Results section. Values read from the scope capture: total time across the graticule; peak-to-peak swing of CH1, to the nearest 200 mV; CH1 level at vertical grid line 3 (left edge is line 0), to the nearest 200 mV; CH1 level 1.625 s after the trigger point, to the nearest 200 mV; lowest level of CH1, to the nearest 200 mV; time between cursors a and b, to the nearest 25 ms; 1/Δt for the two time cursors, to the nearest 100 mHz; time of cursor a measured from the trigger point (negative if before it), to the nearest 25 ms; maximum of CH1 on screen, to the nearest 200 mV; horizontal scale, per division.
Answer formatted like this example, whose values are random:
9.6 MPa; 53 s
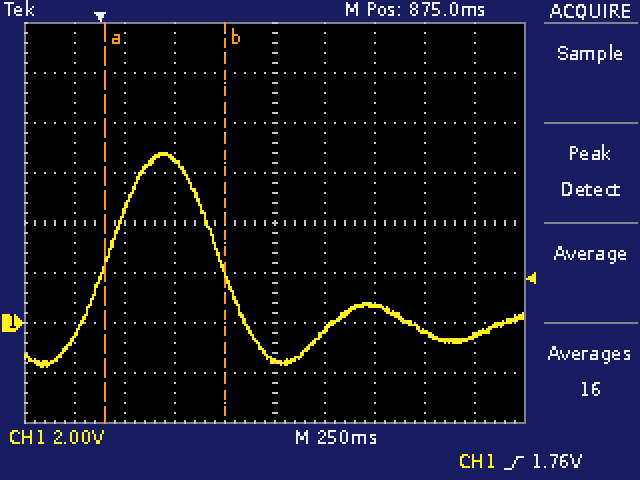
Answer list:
2.5 s; 8.6 V; 6.6 V; -400 mV; -1.8 V; 600 ms; 1.7 Hz; +25 ms; 6.8 V; 250 ms
